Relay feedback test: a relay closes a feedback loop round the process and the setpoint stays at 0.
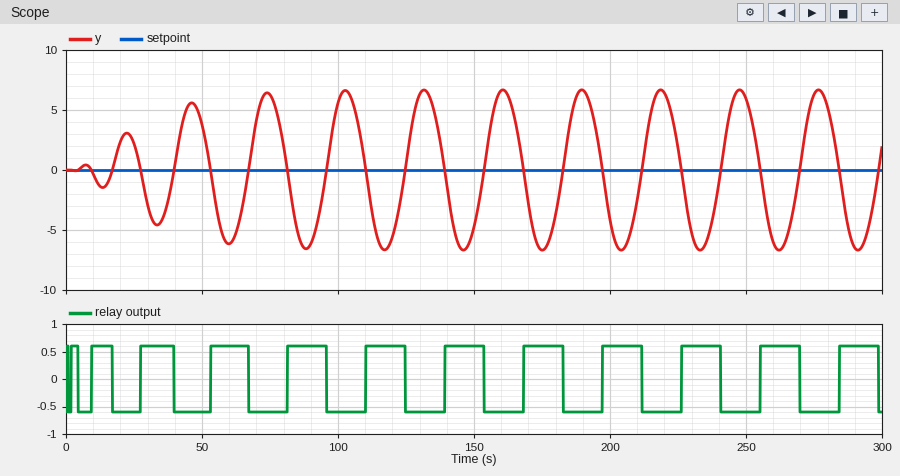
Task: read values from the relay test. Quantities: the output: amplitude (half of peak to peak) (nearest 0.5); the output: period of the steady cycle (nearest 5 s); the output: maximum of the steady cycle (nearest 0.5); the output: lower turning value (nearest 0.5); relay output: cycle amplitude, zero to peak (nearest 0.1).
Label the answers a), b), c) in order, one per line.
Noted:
a) 6.5
b) 30 s
c) 6.5
d) -6.5
e) 0.6
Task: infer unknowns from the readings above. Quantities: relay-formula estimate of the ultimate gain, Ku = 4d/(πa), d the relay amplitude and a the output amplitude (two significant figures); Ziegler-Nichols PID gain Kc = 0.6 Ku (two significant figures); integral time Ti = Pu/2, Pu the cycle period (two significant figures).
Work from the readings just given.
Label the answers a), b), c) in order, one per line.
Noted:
a) 0.12
b) 0.072
c) 15 s
